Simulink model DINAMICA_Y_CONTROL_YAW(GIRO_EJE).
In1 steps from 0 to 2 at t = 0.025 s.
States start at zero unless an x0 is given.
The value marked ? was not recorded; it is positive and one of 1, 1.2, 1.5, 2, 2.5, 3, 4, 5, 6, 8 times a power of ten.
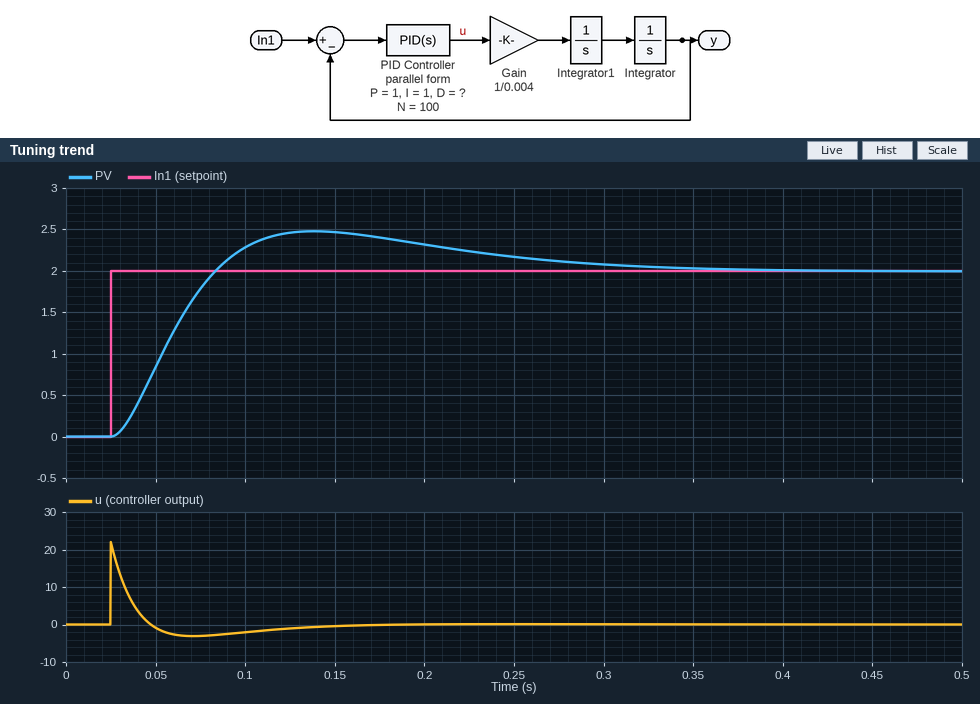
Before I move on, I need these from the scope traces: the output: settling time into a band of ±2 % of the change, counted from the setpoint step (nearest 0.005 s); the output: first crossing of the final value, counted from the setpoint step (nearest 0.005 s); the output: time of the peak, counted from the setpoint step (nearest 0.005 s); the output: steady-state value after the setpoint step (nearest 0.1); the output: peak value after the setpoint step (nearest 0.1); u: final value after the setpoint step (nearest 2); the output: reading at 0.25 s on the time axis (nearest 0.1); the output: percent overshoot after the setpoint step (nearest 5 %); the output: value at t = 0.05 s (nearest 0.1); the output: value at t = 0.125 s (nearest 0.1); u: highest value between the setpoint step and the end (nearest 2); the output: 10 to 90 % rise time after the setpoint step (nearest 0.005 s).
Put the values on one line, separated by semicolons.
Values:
0.310 s; 0.060 s; 0.115 s; 2.0; 2.5; 0; 2.2; 25 %; 0.8; 2.5; 22; 0.040 s
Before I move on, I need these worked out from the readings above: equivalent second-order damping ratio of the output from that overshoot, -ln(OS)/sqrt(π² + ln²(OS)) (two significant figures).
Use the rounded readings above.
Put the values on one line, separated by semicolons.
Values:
0.40
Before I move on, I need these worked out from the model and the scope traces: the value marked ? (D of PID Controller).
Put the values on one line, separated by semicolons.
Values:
0.1
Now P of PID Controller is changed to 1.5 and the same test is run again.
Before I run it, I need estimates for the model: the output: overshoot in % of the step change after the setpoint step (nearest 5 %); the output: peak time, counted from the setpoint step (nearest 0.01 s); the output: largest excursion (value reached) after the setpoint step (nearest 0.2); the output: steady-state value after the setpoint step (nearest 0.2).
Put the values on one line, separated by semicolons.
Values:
30 %; 0.10 s; 2.6; 2.0
